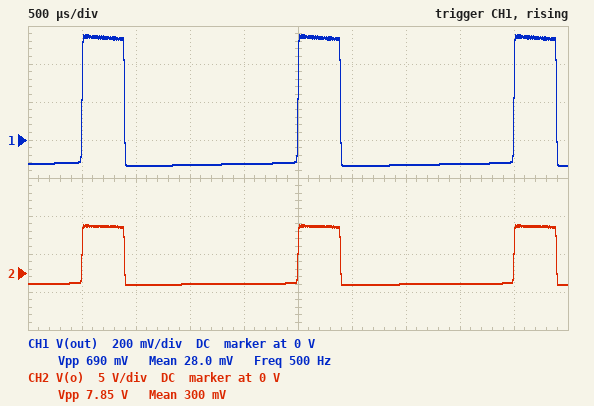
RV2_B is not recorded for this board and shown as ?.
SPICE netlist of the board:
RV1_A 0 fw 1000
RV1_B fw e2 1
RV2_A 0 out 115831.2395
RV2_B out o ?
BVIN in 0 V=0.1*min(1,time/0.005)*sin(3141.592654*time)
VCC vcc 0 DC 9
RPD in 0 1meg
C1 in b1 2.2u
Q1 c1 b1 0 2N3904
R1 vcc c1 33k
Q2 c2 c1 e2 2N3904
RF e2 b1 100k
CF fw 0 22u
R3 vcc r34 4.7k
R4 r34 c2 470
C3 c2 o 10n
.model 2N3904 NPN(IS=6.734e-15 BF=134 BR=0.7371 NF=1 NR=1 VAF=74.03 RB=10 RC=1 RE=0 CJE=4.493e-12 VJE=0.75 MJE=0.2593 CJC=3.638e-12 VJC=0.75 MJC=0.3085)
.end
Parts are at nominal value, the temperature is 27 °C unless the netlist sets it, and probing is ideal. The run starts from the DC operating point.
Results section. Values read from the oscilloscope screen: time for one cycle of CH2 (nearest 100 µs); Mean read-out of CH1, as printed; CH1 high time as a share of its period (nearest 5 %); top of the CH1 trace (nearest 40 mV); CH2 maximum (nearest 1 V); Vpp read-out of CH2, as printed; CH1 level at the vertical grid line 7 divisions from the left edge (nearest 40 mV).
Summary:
2.0 ms
28.0 mV
20 %
560 mV
6 V
7.85 V
-120 mV
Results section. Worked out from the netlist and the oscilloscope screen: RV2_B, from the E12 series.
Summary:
1.2 MΩ
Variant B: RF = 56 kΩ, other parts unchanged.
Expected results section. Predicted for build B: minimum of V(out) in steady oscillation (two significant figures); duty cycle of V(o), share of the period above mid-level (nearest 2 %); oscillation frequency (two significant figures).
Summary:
-150 mV
22 %
500 Hz
